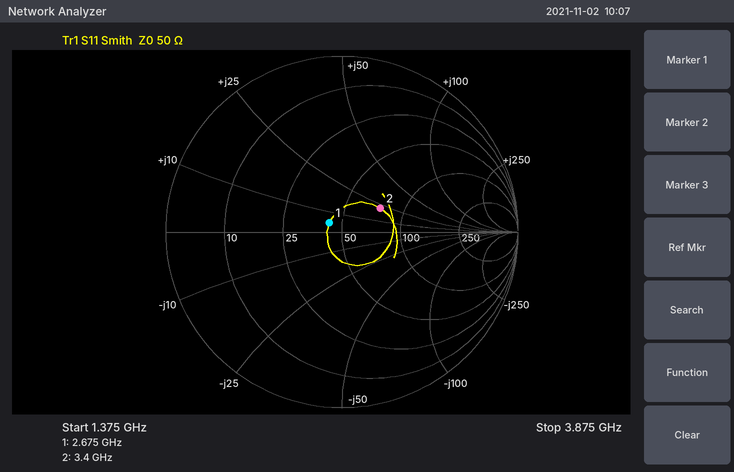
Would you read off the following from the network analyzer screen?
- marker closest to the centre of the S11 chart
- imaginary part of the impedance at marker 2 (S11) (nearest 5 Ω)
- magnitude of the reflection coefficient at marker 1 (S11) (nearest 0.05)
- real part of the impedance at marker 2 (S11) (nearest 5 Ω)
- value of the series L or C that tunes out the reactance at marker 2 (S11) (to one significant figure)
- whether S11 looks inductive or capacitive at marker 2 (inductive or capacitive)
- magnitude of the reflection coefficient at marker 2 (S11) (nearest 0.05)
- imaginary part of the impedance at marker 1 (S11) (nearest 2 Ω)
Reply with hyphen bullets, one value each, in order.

- marker 1
- +20 Ω
- 0.10
- 75 Ω
- 2 pF
- inductive
- 0.25
- +4 Ω
